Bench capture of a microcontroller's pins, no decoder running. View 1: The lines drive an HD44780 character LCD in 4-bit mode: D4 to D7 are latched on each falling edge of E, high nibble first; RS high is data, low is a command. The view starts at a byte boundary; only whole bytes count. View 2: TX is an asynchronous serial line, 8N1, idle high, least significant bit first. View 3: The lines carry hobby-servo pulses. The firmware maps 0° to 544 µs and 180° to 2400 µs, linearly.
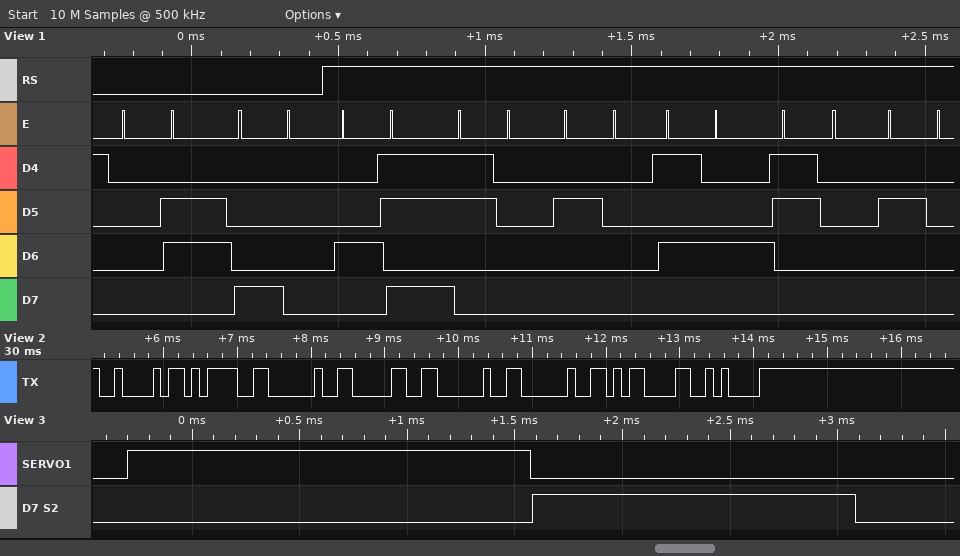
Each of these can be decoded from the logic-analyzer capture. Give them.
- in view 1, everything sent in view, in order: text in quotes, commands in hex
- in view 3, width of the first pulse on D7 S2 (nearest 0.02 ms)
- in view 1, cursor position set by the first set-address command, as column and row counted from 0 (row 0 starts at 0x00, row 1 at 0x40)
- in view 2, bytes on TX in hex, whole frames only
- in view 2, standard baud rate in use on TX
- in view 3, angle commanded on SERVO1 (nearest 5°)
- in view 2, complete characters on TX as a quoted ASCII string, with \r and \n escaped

0x06 0x80 "K0 T0 "
1.50 ms
column 0, row 0
42 3D 20 30 20 20 0D 0A
9600 baud
130°
"B= 0  \r\n"
